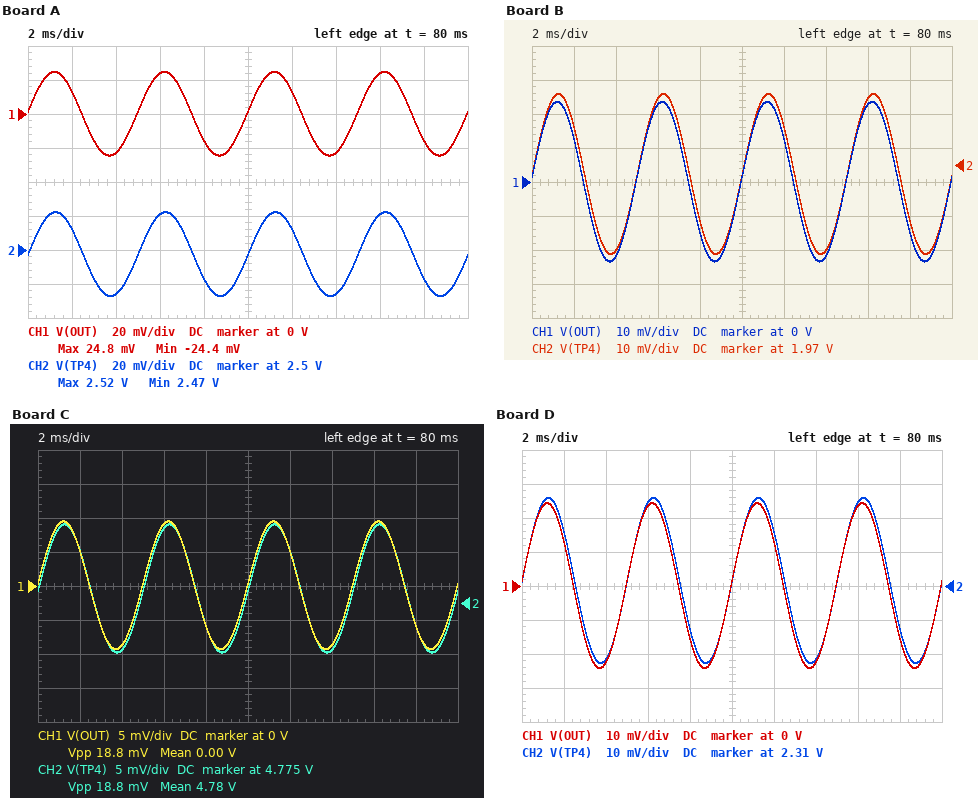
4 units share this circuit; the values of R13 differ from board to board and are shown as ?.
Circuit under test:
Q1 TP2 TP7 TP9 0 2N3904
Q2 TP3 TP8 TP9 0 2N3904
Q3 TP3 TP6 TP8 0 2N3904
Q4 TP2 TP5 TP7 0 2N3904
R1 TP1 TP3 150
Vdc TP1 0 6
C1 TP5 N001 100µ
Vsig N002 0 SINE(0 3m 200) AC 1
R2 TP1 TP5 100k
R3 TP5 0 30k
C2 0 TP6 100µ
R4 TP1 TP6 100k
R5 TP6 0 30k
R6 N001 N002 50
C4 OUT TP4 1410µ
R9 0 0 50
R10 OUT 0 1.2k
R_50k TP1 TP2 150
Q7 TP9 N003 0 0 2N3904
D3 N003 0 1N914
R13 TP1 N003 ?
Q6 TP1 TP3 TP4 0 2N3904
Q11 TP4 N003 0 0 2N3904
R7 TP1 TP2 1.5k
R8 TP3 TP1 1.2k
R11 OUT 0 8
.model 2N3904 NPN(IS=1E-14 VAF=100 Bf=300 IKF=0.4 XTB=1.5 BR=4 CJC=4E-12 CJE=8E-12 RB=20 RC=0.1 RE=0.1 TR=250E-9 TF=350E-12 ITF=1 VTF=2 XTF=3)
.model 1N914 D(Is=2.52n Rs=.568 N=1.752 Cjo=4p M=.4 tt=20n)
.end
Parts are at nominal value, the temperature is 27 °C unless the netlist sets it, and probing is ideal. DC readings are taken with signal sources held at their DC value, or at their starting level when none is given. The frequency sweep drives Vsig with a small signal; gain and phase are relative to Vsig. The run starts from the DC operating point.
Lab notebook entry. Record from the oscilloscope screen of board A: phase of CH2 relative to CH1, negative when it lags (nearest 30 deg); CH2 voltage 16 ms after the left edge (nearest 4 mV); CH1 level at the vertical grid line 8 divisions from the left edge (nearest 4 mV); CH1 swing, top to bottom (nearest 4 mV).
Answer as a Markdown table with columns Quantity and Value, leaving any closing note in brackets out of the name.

| Quantity | Value |
|---|---|
| phase of CH2 relative to CH1, negative when it lags | 0 deg |
| CH2 voltage 16 ms after the left edge | 2.520 V |
| CH1 level at the vertical grid line 8 divisions from the left edge | 24 mV |
| CH1 swing, top to bottom | 48 mV |
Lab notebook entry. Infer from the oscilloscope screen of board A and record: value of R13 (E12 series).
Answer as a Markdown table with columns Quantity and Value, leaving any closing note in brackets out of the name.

| Quantity | Value |
|---|---|
| value of R13 | 82 Ω |
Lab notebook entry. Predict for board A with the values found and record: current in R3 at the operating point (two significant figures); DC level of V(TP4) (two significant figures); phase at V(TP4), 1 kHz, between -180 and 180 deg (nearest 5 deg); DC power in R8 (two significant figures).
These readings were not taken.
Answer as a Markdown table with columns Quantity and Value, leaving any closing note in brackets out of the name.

| Quantity | Value |
|---|---|
| current in R3 at the operating point | 46 µA |
| DC level of V(TP4) | 2.5 V |
| phase at V(TP4), 1 kHz, between -180 and 180 deg | 0 deg |
| DC power in R8 | 6.1 mW |
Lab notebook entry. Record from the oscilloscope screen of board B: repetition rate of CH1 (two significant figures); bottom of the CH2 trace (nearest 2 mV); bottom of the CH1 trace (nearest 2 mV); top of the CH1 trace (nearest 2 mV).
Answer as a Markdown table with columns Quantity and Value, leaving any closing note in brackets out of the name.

| Quantity | Value |
|---|---|
| repetition rate of CH1 | 200 Hz |
| bottom of the CH2 trace | 1.944 V |
| bottom of the CH1 trace | -24 mV |
| top of the CH1 trace | 24 mV |
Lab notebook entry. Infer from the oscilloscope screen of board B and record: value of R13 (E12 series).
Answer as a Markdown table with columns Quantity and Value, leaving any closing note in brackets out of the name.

| Quantity | Value |
|---|---|
| value of R13 | 47 Ω |
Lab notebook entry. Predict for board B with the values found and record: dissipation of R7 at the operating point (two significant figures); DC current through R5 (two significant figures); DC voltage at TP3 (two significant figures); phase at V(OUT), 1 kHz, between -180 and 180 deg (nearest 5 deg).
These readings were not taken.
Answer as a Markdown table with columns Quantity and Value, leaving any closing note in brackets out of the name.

| Quantity | Value |
|---|---|
| dissipation of R7 at the operating point | 6.4 mW |
| DC current through R5 | 46 µA |
| DC voltage at TP3 | 2.8 V |
| phase at V(OUT), 1 kHz, between -180 and 180 deg | 0 deg |
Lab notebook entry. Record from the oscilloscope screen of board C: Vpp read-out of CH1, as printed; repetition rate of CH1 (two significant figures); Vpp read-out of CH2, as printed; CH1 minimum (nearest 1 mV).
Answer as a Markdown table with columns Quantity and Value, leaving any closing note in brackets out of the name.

| Quantity | Value |
|---|---|
| Vpp read-out of CH1, as printed | 18.8 mV |
| repetition rate of CH1 | 200 Hz |
| Vpp read-out of CH2, as printed | 18.8 mV |
| CH1 minimum | -9 mV |
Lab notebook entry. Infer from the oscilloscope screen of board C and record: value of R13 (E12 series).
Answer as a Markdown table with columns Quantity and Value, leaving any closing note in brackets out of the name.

| Quantity | Value |
|---|---|
| value of R13 | 390 Ω |
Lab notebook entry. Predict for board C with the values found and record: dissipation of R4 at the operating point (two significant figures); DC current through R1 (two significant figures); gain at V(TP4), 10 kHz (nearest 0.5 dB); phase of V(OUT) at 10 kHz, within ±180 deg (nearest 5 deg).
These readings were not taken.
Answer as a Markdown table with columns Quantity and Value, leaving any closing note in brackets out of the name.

| Quantity | Value |
|---|---|
| dissipation of R4 at the operating point | 210 µW |
| DC current through R1 | 3.4 mA |
| gain at V(TP4), 10 kHz | 10.0 dB |
| phase of V(OUT) at 10 kHz, within ±180 deg | 0 deg |
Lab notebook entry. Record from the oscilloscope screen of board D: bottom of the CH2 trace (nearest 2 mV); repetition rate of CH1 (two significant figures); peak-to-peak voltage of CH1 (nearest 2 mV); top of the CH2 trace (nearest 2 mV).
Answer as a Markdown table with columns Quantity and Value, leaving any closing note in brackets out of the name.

| Quantity | Value |
|---|---|
| bottom of the CH2 trace | 2.288 V |
| repetition rate of CH1 | 200 Hz |
| peak-to-peak voltage of CH1 | 48 mV |
| top of the CH2 trace | 2.336 V |
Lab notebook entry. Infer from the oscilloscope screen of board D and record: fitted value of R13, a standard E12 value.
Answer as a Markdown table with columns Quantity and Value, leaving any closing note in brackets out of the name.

| Quantity | Value |
|---|---|
| fitted value of R13, a standard E12 value | 68 Ω |
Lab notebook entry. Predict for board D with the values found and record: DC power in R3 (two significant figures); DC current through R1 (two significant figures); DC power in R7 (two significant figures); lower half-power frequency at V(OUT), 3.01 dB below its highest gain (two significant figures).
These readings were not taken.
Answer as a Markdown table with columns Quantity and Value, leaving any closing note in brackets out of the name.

| Quantity | Value |
|---|---|
| DC power in R3 | 63 µW |
| DC current through R1 | 19 mA |
| DC power in R7 | 5.4 mW |
| lower half-power frequency at V(OUT), 3.01 dB below its highest gain | 12 Hz |
